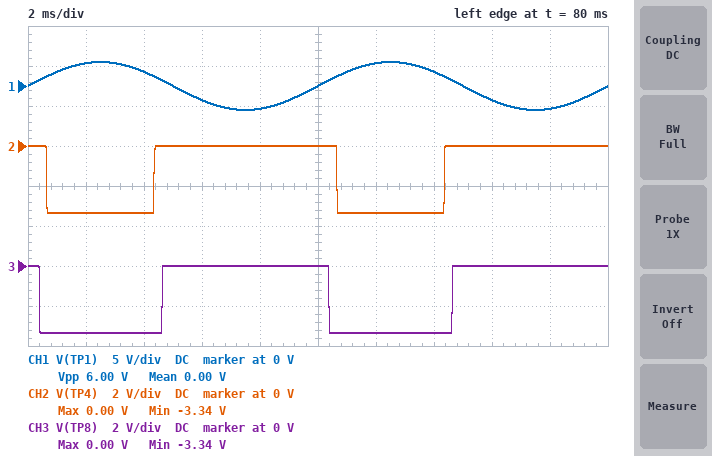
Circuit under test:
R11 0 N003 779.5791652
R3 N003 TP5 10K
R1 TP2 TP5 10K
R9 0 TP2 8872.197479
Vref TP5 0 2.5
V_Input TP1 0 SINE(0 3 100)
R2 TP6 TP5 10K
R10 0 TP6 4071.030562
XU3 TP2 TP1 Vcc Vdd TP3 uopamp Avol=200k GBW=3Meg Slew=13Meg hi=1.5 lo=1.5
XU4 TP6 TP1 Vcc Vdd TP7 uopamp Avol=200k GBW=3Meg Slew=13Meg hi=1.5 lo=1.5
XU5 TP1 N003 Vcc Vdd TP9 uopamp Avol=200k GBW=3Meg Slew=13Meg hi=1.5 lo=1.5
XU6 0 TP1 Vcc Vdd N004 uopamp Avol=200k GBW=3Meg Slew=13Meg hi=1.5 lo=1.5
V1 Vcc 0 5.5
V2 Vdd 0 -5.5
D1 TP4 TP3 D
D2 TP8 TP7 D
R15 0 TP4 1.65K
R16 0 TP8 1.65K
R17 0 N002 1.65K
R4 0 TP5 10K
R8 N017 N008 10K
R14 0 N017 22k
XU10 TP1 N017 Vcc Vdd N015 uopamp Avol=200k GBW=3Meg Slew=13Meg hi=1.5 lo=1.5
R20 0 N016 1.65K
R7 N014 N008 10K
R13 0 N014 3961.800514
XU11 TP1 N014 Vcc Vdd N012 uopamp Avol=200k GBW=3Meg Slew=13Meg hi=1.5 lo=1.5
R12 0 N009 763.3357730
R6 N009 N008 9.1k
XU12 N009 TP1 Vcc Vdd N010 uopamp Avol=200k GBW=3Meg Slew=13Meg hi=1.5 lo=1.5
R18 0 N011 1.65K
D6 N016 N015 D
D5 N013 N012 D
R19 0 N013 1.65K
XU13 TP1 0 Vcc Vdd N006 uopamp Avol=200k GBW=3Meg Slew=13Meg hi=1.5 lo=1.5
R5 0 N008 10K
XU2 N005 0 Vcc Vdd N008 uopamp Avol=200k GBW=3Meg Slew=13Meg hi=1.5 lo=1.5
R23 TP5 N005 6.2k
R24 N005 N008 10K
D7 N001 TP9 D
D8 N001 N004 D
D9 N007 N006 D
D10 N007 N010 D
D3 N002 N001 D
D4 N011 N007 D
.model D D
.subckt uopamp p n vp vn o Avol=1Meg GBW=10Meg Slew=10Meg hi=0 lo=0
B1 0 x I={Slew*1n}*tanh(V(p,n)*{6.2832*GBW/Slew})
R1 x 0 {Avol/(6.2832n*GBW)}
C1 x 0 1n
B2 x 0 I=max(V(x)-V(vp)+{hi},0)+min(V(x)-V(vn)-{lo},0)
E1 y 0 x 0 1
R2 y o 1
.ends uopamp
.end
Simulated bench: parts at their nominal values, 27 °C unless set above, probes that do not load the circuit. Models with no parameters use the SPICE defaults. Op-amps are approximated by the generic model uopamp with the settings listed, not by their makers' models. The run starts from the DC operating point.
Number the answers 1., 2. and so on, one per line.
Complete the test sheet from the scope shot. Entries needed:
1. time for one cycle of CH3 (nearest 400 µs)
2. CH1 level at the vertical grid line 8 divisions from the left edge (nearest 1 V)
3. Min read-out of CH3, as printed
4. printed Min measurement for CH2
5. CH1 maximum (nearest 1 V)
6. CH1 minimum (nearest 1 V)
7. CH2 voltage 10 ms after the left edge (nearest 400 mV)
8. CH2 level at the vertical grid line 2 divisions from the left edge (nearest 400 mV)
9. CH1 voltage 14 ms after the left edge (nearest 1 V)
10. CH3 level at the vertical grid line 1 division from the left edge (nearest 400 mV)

1. 10.0 ms
2. -2 V
3. -3.34 V
4. -3.34 V
5. 3 V
6. -3 V
7. 0 V
8. -3.2 V
9. 2 V
10. -3.2 V
